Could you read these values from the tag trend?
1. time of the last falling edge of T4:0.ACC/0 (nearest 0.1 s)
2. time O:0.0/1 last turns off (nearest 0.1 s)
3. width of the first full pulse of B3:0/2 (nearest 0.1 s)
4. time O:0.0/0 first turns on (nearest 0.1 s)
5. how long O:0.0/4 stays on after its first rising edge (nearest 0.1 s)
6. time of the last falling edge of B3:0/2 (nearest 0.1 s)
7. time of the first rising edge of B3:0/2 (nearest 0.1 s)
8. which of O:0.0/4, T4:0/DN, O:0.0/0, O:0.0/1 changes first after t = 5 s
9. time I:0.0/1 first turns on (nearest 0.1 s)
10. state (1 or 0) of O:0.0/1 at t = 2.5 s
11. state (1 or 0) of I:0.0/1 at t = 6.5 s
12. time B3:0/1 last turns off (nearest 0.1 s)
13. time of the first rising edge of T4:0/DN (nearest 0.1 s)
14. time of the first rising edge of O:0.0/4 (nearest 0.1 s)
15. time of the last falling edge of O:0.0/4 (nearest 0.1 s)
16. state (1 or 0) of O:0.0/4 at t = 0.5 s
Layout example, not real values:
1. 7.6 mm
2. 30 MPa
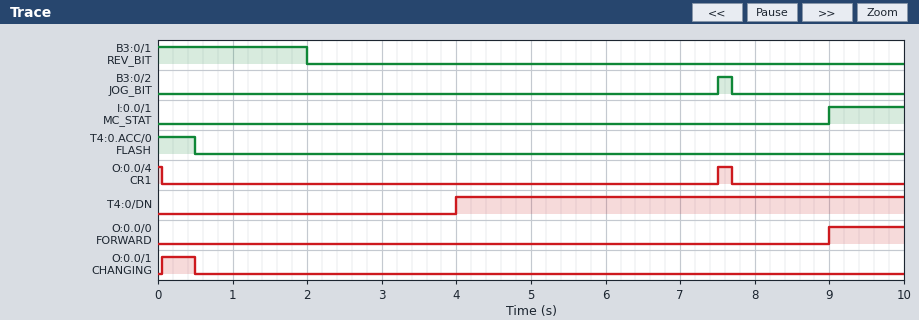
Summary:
1. 0.5 s
2. 0.5 s
3. 0.2 s
4. 9.0 s
5. 0.2 s
6. 7.7 s
7. 7.5 s
8. O:0.0/4
9. 9.0 s
10. 0
11. 0
12. 2.0 s
13. 4.0 s
14. 7.5 s
15. 7.7 s
16. 0
